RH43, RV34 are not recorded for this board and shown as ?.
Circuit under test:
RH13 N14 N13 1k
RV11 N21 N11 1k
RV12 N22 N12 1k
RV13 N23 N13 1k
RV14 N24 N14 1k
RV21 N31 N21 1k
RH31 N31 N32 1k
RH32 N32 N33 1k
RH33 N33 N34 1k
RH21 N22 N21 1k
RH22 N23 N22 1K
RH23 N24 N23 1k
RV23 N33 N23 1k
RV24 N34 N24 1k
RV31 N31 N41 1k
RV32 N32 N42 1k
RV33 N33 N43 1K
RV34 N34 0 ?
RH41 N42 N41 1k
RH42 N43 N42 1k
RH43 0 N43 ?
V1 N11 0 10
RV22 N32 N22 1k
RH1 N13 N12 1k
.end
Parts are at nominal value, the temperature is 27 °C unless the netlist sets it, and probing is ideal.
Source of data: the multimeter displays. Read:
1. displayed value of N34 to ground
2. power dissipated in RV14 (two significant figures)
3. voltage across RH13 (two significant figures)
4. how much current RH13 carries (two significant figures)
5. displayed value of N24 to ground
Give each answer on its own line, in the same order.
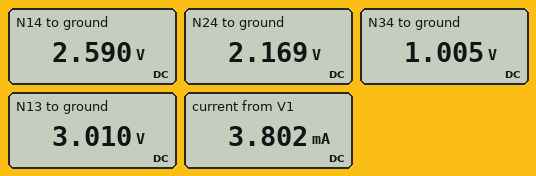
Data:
1.005 V
180 µW
420 mV
420 µA
2.169 V
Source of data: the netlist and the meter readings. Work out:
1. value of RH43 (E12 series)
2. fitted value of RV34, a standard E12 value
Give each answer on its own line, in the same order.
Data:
1.8 kΩ
390 Ω
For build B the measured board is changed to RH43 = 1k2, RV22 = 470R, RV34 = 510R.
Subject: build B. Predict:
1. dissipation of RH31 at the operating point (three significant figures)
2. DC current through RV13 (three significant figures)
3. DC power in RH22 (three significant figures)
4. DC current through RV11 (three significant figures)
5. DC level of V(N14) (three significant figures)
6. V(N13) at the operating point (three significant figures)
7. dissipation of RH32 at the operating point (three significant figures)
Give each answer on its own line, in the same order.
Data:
875 µW
95.8 µA
1.09 mW
3.87 mA
2.57 V
2.95 V
1.41 mW
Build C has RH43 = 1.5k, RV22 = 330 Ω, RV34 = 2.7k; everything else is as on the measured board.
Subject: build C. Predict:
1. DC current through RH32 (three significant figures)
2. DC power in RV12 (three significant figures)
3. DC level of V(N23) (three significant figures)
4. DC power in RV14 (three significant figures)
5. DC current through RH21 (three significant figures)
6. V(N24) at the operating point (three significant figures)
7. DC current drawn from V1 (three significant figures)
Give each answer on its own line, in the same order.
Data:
933 µA
107 µW
4.24 V
56.6 µW
1.83 mA
3.85 V
3.19 mA
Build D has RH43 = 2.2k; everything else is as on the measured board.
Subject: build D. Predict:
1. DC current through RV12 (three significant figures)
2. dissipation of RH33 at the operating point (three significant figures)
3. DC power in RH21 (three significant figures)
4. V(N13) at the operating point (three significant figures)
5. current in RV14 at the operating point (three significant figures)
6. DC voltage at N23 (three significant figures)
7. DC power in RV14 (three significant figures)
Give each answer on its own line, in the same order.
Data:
521 µA
2.18 mW
4.53 mW
3.08 V
427 µA
2.99 V
182 µW
